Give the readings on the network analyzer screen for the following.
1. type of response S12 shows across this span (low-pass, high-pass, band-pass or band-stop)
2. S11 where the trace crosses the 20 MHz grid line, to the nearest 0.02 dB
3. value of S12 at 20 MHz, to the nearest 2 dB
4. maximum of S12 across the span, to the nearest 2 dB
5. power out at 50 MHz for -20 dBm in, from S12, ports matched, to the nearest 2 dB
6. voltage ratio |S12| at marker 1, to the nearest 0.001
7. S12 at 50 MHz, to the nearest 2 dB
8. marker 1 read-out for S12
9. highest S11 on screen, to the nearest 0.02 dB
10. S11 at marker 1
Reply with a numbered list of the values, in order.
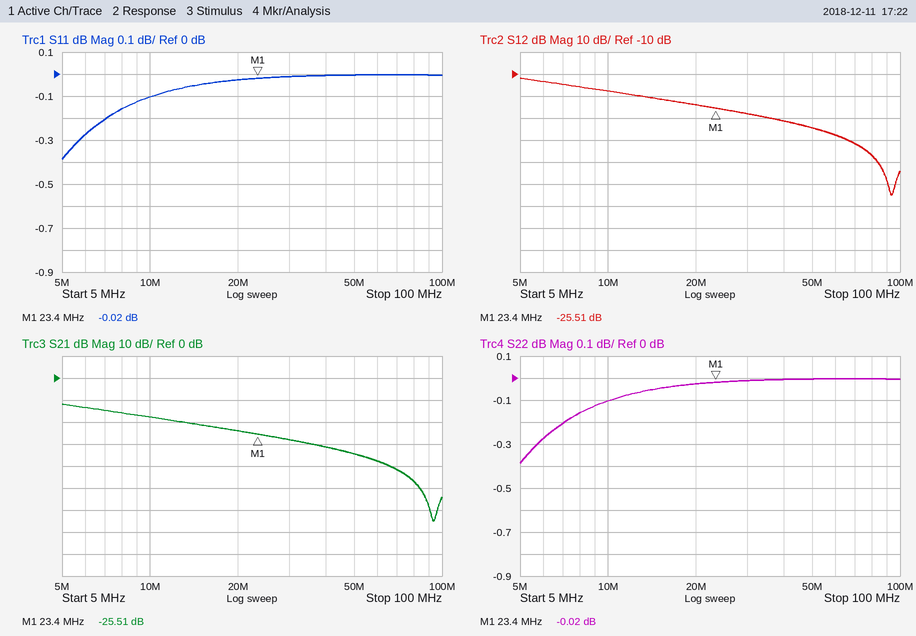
1. low-pass
2. -0.02 dB
3. -24 dB
4. -12 dB
5. -54 dBm
6. 0.053
7. -34 dB
8. -25.51 dB
9. 0.00 dB
10. -0.02 dB
